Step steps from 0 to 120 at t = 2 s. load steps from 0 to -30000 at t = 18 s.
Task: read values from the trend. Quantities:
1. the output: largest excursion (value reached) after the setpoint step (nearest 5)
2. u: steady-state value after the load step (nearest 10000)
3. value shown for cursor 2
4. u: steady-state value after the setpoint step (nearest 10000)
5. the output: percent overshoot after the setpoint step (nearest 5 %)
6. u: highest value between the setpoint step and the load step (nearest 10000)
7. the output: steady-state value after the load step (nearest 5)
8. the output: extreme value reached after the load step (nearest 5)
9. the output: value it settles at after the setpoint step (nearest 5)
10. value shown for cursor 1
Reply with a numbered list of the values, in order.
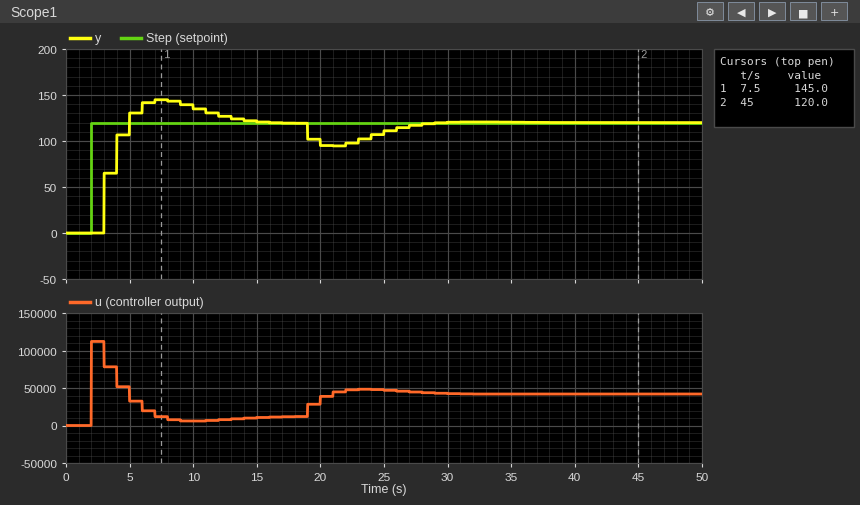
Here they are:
1. 145
2. 40000
3. 120.0
4. 10000
5. 20 %
6. 110000
7. 120
8. 95
9. 120
10. 145.0
